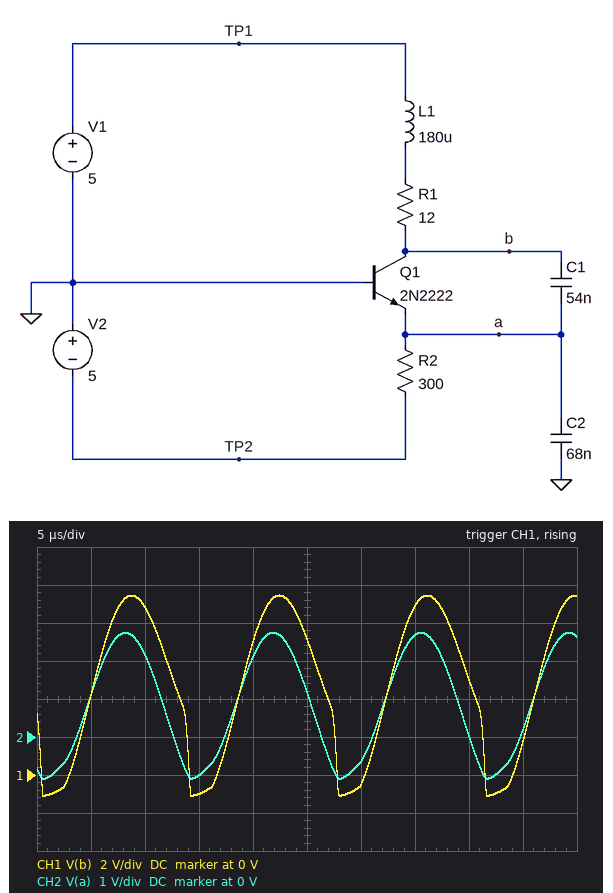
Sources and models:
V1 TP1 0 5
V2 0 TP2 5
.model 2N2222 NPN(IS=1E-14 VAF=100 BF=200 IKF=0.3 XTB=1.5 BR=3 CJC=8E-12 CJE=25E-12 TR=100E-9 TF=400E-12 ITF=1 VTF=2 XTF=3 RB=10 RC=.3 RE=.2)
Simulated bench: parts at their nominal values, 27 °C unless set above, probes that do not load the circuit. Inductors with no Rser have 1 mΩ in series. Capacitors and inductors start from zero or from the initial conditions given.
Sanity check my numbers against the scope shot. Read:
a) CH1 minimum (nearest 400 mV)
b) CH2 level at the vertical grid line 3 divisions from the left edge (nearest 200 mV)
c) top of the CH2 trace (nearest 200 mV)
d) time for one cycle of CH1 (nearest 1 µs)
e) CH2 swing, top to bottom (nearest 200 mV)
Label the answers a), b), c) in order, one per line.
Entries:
a) -1.2 V
b) -1.0 V
c) 2.8 V
d) 14 µs
e) 3.8 V
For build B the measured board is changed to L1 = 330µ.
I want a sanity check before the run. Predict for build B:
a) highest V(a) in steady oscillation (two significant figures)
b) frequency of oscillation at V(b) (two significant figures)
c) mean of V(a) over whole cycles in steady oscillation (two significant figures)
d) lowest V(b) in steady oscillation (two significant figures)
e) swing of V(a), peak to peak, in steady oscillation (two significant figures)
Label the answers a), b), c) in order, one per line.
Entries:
a) 2.5 V
b) 56 kHz
c) 710 mV
d) -1.1 V
e) 3.6 V
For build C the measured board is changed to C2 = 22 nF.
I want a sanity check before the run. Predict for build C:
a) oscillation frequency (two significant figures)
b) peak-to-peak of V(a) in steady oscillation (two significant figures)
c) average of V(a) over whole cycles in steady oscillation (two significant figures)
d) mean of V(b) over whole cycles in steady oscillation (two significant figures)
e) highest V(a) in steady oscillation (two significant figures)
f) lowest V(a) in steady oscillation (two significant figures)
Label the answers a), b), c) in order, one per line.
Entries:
a) 98 kHz
b) 5.5 V
c) 1.8 V
d) 4.7 V
e) 4.5 V
f) -1.0 V
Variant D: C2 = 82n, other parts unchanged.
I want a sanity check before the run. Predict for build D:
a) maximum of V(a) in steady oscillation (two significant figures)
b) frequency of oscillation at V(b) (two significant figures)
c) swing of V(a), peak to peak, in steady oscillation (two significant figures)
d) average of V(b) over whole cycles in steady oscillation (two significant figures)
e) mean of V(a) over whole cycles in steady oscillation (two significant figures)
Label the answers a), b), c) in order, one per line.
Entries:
a) 2.4 V
b) 70 kHz
c) 3.5 V
d) 4.8 V
e) 710 mV
